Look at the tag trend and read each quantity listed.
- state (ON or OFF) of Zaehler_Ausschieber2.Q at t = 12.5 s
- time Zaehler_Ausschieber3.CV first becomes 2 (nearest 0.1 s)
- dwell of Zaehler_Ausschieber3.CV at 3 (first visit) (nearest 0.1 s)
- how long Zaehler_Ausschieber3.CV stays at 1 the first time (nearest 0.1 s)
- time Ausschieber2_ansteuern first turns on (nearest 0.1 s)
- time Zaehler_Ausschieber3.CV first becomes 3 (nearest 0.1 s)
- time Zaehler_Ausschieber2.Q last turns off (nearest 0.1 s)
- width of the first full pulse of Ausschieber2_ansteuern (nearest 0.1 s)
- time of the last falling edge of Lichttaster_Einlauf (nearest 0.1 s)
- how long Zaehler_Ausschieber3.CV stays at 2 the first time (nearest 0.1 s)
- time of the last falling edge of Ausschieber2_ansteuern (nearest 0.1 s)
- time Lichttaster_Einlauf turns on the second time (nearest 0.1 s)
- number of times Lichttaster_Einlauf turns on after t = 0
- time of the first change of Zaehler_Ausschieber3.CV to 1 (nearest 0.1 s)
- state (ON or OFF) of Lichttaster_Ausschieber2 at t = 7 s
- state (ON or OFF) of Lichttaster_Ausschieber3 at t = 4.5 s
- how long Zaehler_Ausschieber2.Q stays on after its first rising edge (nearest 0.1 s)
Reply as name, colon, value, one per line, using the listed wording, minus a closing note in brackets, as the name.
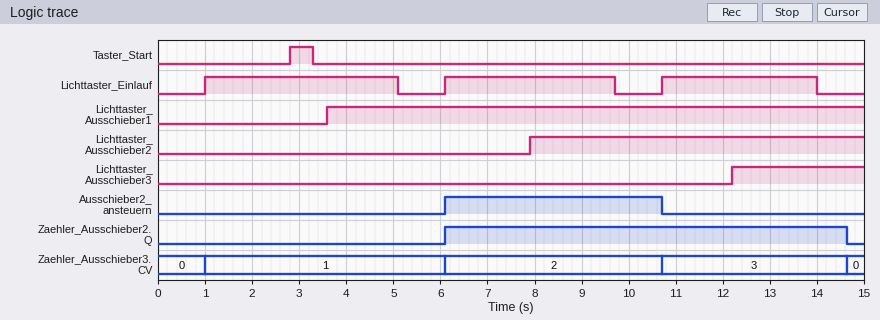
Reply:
state (ON or OFF) of Zaehler_Ausschieber2.Q at t = 12.5 s: ON
time Zaehler_Ausschieber3.CV first becomes 2: 6.1 s
dwell of Zaehler_Ausschieber3.CV at 3 (first visit): 3.9 s
how long Zaehler_Ausschieber3.CV stays at 1 the first time: 5.1 s
time Ausschieber2_ansteuern first turns on: 6.1 s
time Zaehler_Ausschieber3.CV first becomes 3: 10.7 s
time Zaehler_Ausschieber2.Q last turns off: 14.6 s
width of the first full pulse of Ausschieber2_ansteuern: 4.6 s
time of the last falling edge of Lichttaster_Einlauf: 14.0 s
how long Zaehler_Ausschieber3.CV stays at 2 the first time: 4.6 s
time of the last falling edge of Ausschieber2_ansteuern: 10.7 s
time Lichttaster_Einlauf turns on the second time: 6.1 s
number of times Lichttaster_Einlauf turns on after t = 0: 3
time of the first change of Zaehler_Ausschieber3.CV to 1: 1.0 s
state (ON or OFF) of Lichttaster_Ausschieber2 at t = 7 s: OFF
state (ON or OFF) of Lichttaster_Ausschieber3 at t = 4.5 s: OFF
how long Zaehler_Ausschieber2.Q stays on after its first rising edge: 8.5 s
